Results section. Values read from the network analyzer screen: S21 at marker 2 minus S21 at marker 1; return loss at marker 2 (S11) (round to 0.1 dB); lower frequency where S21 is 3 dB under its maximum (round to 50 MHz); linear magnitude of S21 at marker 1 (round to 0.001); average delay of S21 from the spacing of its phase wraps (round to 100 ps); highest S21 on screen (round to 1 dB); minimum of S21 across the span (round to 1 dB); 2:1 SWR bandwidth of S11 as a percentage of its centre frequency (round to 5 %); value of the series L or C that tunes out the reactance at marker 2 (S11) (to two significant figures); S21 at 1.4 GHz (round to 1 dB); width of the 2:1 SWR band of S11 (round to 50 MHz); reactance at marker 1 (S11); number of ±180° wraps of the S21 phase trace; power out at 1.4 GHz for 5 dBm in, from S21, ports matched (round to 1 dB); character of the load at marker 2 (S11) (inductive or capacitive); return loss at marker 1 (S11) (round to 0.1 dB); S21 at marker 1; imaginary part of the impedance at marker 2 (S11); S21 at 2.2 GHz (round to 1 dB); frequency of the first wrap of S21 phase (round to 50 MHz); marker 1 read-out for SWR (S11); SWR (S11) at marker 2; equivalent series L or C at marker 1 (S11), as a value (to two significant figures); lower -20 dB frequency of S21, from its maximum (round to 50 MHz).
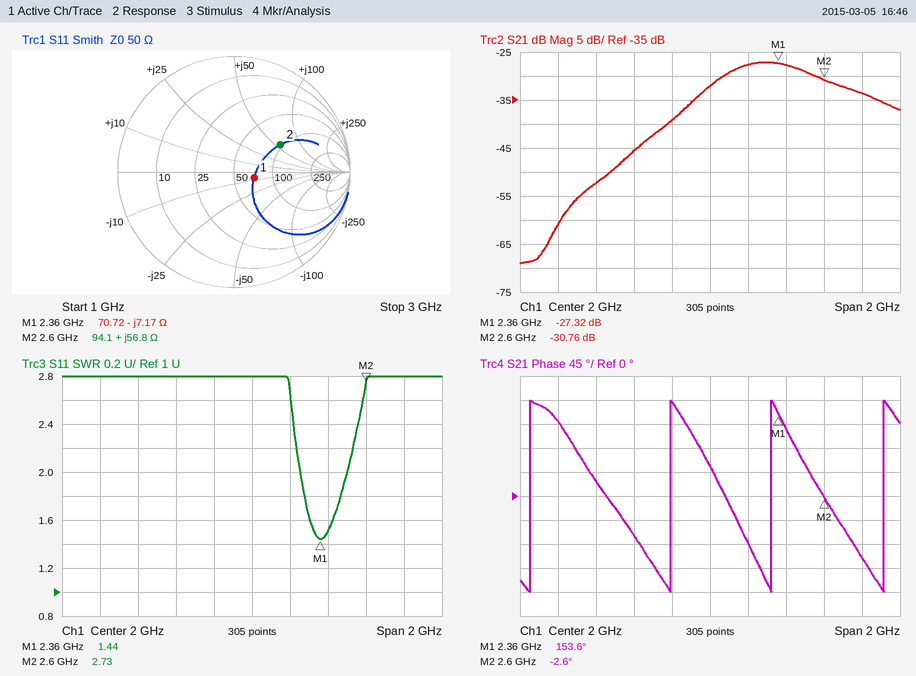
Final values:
-3.44 dB
6.7 dB
2.05 GHz
0.043
1.6 ns
-27 dB
-69 dB
10 %
1.1 pF
-52 dB
250 MHz
-7.17 Ω
4
-47 dBm
inductive
14.8 dB
-27.32 dB
+56.8 Ω
-28 dB
1.05 GHz
1.44
2.73
9.4 pF
1.55 GHz
